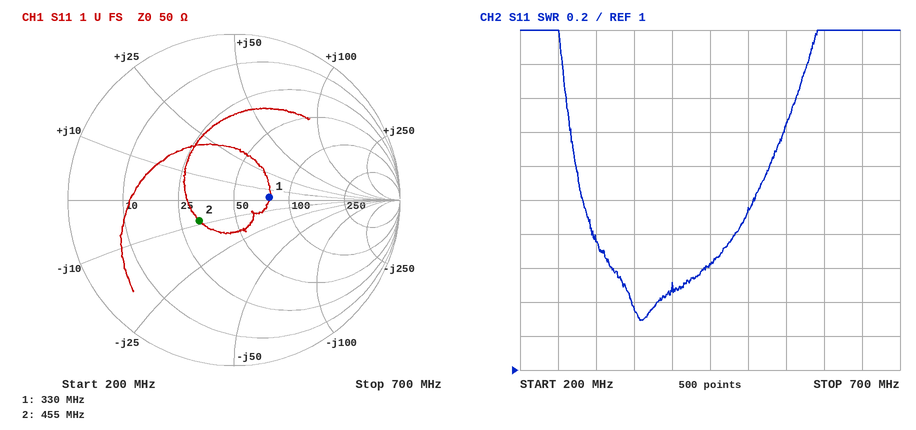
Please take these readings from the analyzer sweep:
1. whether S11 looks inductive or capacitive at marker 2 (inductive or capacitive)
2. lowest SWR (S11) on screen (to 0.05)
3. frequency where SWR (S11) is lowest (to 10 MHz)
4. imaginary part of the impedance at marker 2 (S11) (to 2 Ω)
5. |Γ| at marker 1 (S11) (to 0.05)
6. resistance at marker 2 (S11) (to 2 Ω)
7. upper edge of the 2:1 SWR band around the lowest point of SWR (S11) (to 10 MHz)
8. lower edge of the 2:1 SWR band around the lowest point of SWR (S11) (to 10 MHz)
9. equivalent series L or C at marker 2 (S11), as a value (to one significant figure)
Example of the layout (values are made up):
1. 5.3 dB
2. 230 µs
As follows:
1. capacitive
2. 1.30
3. 360 MHz
4. -8 Ω
5. 0.20
6. 32 Ω
7. 510 MHz
8. 280 MHz
9. 40 pF
